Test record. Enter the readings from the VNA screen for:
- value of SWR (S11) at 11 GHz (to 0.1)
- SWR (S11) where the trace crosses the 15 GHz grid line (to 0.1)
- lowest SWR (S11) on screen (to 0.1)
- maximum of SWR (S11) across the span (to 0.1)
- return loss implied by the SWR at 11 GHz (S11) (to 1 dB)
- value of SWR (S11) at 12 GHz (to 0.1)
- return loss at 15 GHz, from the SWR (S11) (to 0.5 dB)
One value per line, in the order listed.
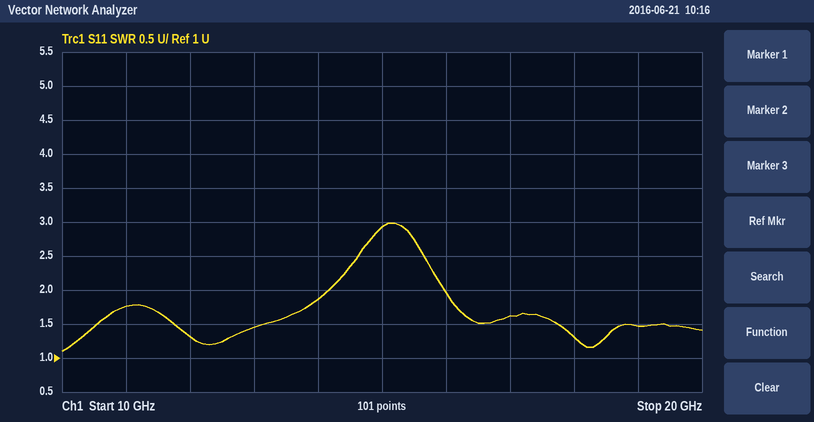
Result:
1.8
2.9
1.1
3.0
11 dB
1.3
6.0 dB
